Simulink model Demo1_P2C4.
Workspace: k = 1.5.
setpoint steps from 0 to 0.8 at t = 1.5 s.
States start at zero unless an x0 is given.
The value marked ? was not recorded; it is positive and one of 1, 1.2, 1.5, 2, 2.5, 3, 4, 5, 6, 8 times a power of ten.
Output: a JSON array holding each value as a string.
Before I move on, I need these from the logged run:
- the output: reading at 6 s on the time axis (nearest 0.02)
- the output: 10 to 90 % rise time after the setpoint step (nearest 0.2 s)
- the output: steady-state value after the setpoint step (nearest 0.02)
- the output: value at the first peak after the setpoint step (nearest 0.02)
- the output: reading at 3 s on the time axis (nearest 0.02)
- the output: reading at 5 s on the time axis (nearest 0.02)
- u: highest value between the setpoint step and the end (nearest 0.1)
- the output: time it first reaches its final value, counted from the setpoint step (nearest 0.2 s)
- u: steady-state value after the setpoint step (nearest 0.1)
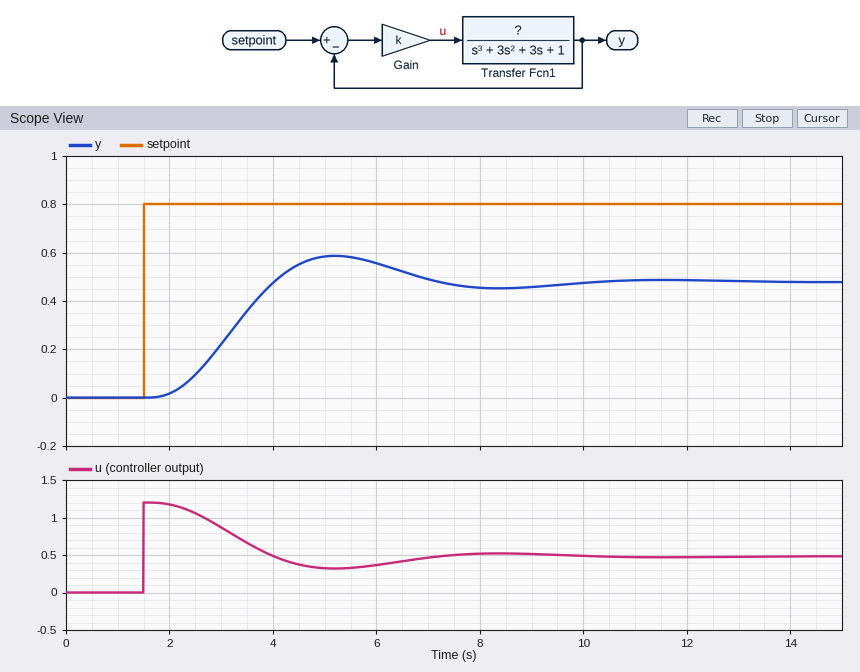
["0.56", "1.6 s", "0.48", "0.58", "0.22", "0.58", "1.2", "2.6 s", "0.5"]
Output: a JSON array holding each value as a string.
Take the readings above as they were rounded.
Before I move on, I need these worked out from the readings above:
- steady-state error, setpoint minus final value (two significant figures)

["0.32"]
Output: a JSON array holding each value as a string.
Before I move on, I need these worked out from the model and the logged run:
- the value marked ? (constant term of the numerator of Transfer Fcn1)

["1"]
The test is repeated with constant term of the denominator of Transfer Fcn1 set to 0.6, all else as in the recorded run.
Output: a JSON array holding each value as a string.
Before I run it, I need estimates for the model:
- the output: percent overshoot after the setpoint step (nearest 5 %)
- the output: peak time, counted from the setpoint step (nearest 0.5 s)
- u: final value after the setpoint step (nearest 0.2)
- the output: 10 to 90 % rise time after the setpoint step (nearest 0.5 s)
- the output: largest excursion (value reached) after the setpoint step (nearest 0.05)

["15 %", "4.0 s", "0.4", "2.0 s", "0.65"]
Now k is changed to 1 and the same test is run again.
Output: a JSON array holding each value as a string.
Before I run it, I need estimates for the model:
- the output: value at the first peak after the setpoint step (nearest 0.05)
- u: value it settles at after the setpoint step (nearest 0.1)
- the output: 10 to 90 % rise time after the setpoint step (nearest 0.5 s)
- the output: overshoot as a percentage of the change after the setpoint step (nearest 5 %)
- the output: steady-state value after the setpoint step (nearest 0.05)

["0.45", "0.4", "2.0 s", "15 %", "0.40"]
